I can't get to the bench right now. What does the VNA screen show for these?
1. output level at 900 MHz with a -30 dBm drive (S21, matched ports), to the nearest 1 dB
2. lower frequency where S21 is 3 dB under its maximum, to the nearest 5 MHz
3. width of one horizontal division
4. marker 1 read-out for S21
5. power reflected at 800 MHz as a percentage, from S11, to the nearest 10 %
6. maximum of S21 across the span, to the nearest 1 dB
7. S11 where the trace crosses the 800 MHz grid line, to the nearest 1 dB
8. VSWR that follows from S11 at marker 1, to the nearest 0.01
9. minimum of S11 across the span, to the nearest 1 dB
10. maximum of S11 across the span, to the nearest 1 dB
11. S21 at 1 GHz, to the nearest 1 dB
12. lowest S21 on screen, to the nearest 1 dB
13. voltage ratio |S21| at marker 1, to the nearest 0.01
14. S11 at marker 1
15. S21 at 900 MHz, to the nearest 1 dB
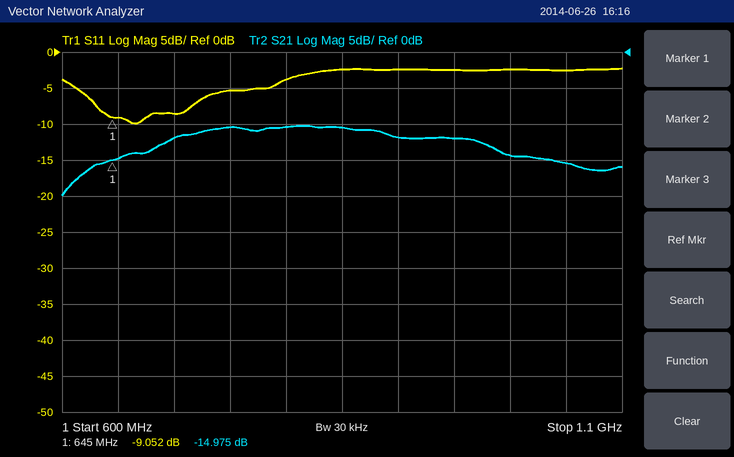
-42 dBm
685 MHz
50 MHz
-14.975 dB
40 %
-10 dB
-4 dB
2.09
-10 dB
-2 dB
-14 dB
-20 dB
0.18
-9.052 dB
-12 dB
